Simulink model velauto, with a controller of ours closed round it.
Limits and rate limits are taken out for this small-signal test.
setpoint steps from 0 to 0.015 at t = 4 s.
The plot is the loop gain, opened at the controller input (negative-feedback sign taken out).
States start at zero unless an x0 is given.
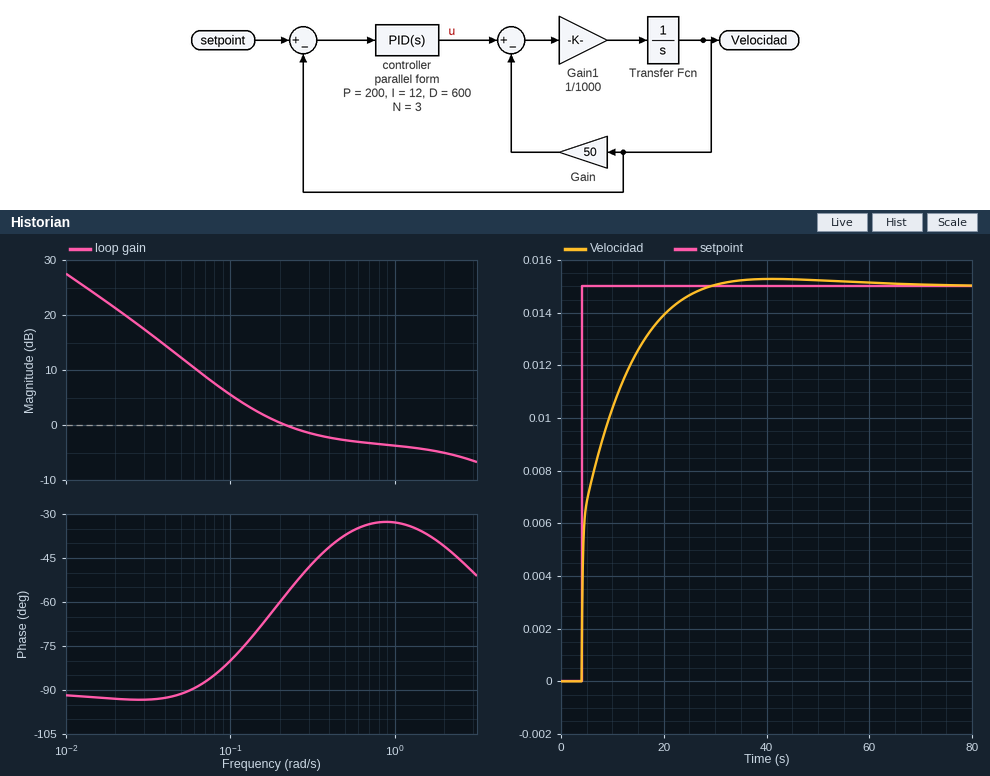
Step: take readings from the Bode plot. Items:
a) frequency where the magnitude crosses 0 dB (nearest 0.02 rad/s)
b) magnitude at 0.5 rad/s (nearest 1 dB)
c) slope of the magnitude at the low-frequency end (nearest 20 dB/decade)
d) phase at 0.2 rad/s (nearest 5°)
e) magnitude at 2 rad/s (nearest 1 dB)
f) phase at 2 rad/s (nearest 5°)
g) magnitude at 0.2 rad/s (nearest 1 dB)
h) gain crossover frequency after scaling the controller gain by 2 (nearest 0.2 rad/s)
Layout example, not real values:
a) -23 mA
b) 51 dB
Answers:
a) 0.22 rad/s
b) -3 dB
c) -20 dB/decade
d) -60°
e) -5 dB
f) -40°
g) 0 dB
h) 2.6 rad/s
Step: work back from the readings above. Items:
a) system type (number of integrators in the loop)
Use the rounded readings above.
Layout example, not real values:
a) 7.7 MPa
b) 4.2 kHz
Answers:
a) 1
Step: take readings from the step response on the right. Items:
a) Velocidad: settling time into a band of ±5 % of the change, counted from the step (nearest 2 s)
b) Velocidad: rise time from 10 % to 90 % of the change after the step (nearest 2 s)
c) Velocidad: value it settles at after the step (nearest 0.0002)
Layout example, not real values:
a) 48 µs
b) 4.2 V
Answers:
a) 18 s
b) 14 s
c) 0.0150
